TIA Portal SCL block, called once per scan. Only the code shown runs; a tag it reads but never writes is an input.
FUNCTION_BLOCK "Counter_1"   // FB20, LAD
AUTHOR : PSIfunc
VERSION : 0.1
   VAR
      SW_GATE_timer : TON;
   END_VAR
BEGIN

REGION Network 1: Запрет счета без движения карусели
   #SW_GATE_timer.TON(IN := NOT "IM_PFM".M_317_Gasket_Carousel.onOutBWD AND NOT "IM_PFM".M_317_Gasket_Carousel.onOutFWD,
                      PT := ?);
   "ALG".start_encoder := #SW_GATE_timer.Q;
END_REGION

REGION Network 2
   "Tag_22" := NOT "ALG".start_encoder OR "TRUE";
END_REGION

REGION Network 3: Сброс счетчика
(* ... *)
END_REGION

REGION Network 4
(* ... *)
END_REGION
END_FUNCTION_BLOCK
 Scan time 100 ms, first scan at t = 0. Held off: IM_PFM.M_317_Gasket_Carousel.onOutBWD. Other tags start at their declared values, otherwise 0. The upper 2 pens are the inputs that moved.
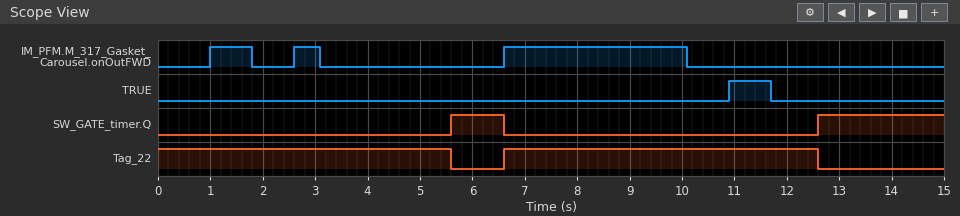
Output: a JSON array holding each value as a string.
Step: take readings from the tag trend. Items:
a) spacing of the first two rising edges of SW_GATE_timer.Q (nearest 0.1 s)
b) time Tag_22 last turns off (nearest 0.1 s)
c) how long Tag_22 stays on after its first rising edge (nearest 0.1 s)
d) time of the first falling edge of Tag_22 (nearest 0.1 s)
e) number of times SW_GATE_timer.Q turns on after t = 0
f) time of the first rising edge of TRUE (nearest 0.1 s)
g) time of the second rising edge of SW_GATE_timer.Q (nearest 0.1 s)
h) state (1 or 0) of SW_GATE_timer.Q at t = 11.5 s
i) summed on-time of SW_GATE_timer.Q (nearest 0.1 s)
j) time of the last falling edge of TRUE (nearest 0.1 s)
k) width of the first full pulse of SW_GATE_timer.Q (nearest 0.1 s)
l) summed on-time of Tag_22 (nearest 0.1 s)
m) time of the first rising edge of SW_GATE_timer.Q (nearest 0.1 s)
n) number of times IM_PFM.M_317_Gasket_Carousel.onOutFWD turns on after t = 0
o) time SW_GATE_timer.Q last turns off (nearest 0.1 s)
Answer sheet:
["7.0 s", "12.6 s", "6.0 s", "5.6 s", "2", "10.9 s", "12.6 s", "0", "3.4 s", "11.7 s", "1.0 s", "11.6 s", "5.6 s", "3", "6.6 s"]
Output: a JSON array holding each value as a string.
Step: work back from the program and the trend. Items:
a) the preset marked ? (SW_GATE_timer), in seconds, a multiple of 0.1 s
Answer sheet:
["2.5 s"]
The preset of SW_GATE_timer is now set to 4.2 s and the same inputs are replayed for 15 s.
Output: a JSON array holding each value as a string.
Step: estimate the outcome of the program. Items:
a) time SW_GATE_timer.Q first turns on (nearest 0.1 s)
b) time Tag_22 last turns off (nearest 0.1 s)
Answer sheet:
["14.3 s", "14.3 s"]
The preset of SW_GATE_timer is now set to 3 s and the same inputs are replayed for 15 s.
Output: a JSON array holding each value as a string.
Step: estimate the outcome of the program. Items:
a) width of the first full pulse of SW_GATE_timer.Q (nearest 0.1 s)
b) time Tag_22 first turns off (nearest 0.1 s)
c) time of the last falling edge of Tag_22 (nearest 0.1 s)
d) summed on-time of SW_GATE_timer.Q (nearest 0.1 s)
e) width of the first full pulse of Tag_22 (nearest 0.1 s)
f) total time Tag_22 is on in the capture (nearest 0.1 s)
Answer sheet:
["0.5 s", "6.1 s", "13.1 s", "2.4 s", "6.5 s", "12.6 s"]
